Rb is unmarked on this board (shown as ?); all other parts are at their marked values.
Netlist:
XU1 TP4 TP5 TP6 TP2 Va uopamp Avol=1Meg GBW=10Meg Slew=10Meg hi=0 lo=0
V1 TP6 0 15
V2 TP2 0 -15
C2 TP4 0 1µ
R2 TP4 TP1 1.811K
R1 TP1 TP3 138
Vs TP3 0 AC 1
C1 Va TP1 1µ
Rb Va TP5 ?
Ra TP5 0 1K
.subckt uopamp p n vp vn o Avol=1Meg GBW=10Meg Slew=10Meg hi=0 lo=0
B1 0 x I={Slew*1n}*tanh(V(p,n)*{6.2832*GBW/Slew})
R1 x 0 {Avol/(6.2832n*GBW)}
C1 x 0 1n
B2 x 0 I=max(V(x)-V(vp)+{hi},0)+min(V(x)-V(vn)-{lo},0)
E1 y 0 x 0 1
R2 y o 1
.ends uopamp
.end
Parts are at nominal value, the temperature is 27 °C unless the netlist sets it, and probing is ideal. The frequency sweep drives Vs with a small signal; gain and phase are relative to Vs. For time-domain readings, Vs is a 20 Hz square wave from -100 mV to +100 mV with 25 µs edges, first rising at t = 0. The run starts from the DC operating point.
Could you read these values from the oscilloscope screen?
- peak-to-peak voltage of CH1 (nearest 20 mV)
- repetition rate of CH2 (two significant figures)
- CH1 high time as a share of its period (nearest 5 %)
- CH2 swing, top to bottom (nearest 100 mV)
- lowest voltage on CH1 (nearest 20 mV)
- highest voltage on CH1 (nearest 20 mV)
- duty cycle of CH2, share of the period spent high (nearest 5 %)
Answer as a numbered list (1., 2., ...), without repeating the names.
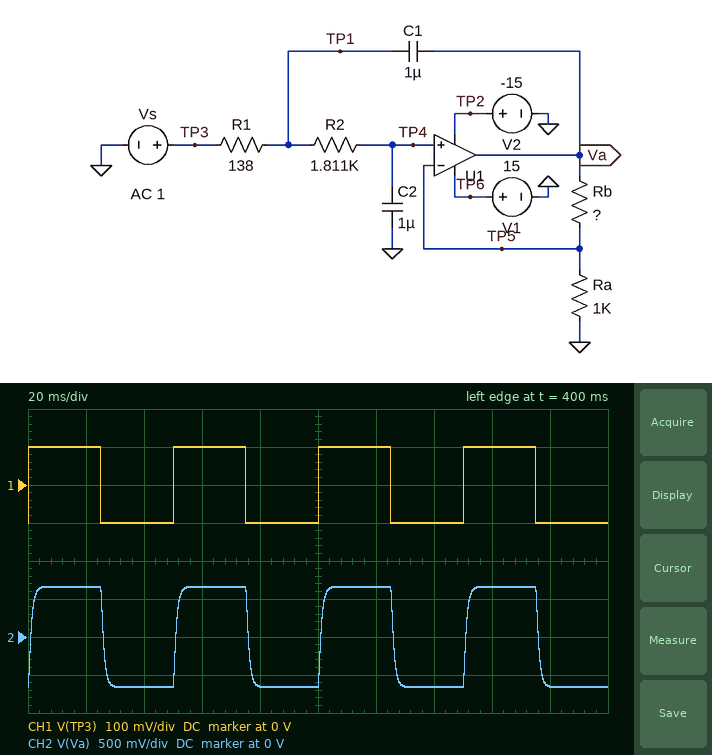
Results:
1. 200 mV
2. 20 Hz
3. 50 %
4. 1.3 V
5. -100 mV
6. 100 mV
7. 50 %
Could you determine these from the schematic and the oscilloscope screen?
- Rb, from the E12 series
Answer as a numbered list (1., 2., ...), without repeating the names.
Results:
1. 5.6 kΩ
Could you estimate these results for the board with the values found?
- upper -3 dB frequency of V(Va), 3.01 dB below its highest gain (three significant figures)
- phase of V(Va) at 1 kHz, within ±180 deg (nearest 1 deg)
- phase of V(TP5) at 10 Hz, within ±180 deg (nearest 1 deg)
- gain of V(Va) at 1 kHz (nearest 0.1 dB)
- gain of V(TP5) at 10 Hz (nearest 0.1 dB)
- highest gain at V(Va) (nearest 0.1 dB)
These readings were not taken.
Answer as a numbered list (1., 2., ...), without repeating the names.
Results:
1. 163 Hz
2. -140 deg
3. -4 deg
4. -4.9 dB
5. 0 dB
6. 16.4 dB
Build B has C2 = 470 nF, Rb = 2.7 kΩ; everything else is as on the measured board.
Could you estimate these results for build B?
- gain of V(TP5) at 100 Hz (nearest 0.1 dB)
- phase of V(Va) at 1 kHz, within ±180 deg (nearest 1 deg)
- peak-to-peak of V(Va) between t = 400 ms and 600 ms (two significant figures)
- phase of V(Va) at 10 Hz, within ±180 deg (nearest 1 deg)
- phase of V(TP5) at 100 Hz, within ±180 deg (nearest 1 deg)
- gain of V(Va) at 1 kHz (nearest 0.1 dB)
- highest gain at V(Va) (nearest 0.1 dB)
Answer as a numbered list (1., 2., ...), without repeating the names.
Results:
1. -0.1 dB
2. -137 deg
3. 770 mV
4. -2 deg
5. -20 deg
6. -2.6 dB
7. 11.4 dB
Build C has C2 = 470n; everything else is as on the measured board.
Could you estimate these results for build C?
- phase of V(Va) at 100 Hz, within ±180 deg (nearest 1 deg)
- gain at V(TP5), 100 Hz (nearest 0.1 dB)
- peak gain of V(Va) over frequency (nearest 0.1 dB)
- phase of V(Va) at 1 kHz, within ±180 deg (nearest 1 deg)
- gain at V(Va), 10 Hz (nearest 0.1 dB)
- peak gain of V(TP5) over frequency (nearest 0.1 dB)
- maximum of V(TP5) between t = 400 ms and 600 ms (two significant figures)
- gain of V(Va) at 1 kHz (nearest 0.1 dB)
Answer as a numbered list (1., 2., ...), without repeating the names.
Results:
1. -5 deg
2. 0.4 dB
3. 24.2 dB
4. -166 deg
5. 16.4 dB
6. 7.8 dB
7. 200 mV
8. 4.9 dB
